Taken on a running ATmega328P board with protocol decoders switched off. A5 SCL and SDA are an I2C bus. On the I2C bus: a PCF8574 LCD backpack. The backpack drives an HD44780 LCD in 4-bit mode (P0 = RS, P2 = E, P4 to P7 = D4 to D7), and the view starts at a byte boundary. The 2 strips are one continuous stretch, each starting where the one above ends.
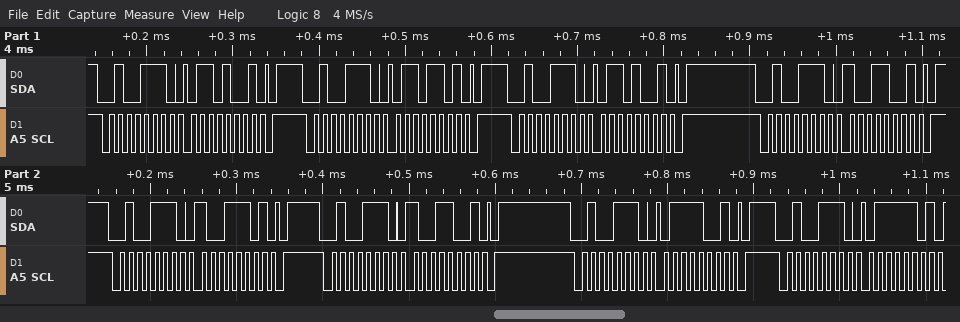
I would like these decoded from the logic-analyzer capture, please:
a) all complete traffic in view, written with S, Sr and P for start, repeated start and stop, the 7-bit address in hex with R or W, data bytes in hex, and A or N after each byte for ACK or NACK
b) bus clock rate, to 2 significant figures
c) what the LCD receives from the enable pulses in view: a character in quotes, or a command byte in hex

S 27W A 69 A P S 27W A 6D A P S 27W A 69 A P S 27W A 99 A P S 27W A 9D A P S 27W A 99 A P S 27W A 79 A P S 27W A 7D A
100 kHz
'i'
